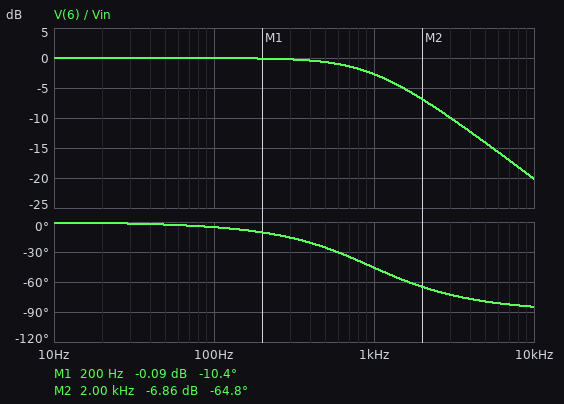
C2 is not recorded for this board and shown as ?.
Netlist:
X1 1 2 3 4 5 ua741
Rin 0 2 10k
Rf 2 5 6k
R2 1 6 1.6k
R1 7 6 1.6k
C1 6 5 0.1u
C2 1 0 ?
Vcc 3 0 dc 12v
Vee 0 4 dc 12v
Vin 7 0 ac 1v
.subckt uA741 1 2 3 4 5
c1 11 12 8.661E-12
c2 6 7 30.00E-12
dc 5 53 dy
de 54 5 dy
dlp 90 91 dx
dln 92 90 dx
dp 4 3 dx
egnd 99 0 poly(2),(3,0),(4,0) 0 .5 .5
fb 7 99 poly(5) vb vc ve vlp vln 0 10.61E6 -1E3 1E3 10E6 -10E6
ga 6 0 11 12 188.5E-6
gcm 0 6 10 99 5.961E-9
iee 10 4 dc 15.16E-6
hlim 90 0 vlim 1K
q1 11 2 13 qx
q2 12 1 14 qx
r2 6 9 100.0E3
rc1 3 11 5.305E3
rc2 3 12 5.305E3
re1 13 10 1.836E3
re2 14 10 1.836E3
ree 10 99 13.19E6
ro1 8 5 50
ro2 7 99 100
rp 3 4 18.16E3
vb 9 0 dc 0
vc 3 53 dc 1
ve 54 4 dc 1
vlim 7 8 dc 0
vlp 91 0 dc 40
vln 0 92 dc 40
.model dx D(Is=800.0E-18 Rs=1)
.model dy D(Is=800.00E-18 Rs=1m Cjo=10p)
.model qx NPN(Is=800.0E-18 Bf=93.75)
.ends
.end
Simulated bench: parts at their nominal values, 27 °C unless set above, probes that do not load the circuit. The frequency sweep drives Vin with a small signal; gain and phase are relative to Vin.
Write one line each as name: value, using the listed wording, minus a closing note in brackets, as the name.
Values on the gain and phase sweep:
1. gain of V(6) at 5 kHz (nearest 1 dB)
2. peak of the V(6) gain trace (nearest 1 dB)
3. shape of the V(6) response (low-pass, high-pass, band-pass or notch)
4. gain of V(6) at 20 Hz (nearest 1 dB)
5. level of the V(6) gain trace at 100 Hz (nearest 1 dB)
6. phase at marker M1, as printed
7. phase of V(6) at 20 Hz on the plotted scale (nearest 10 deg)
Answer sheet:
gain of V(6) at 5 kHz: -14 dB
peak of the V(6) gain trace: 0 dB
shape of the V(6) response: low-pass
gain of V(6) at 20 Hz: 0 dB
level of the V(6) gain trace at 100 Hz: 0 dB
phase at marker M1, as printed: -10.4 deg
phase of V(6) at 20 Hz on the plotted scale: 0 deg
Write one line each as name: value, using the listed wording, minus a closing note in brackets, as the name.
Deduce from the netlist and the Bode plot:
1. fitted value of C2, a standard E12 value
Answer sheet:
fitted value of C2, a standard E12 value: 150 nF
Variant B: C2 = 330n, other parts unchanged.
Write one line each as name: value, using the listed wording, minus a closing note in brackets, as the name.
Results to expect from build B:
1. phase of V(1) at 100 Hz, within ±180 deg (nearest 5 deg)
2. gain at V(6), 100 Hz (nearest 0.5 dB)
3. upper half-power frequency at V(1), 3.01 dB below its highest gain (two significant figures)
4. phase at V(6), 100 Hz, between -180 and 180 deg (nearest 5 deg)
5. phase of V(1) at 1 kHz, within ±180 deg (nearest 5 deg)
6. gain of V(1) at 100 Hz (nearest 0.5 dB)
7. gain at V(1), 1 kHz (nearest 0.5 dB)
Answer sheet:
phase of V(1) at 100 Hz, within ±180 deg: -30 deg
gain at V(6), 100 Hz: -0.5 dB
upper half-power frequency at V(1), 3.01 dB below its highest gain: 180 Hz
phase at V(6), 100 Hz, between -180 and 180 deg: -15 deg
phase of V(1) at 1 kHz, within ±180 deg: -110 deg
gain of V(1) at 100 Hz: -1.0 dB
gain at V(1), 1 kHz: -16.0 dB
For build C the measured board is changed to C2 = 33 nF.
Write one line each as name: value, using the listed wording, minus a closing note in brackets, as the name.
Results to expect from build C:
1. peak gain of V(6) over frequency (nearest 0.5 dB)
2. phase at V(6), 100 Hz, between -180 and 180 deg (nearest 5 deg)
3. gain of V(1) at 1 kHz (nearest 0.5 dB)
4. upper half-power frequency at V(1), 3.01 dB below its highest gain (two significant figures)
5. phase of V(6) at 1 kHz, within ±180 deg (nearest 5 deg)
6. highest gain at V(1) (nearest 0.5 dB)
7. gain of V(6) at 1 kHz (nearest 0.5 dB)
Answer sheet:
peak gain of V(6) over frequency: 21.0 dB
phase at V(6), 100 Hz, between -180 and 180 deg: 0 deg
gain of V(1) at 1 kHz: 3.5 dB
upper half-power frequency at V(1), 3.01 dB below its highest gain: 1.8 kHz
phase of V(6) at 1 kHz, within ±180 deg: 15 deg
highest gain at V(1): 19.5 dB
gain of V(6) at 1 kHz: 4.0 dB
